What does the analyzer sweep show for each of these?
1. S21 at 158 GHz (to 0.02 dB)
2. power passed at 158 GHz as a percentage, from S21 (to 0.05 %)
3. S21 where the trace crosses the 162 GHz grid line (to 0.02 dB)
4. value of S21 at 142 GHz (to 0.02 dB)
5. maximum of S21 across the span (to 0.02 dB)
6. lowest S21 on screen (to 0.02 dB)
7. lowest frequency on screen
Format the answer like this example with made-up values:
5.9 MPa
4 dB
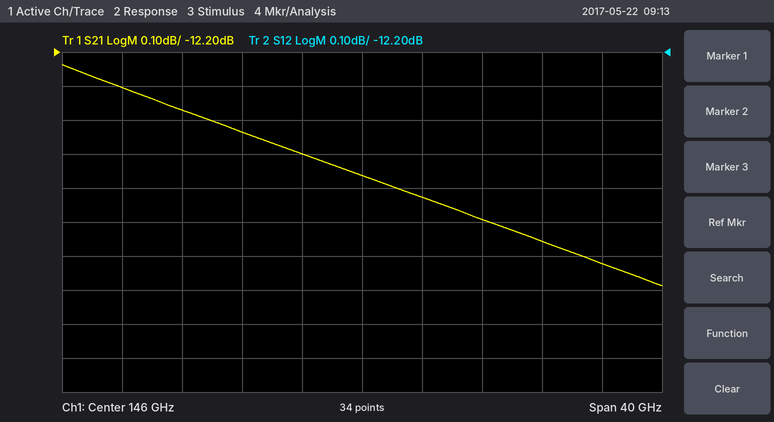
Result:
-12.76 dB
5.30 %
-12.82 dB
-12.50 dB
-12.24 dB
-12.88 dB
126 GHz
